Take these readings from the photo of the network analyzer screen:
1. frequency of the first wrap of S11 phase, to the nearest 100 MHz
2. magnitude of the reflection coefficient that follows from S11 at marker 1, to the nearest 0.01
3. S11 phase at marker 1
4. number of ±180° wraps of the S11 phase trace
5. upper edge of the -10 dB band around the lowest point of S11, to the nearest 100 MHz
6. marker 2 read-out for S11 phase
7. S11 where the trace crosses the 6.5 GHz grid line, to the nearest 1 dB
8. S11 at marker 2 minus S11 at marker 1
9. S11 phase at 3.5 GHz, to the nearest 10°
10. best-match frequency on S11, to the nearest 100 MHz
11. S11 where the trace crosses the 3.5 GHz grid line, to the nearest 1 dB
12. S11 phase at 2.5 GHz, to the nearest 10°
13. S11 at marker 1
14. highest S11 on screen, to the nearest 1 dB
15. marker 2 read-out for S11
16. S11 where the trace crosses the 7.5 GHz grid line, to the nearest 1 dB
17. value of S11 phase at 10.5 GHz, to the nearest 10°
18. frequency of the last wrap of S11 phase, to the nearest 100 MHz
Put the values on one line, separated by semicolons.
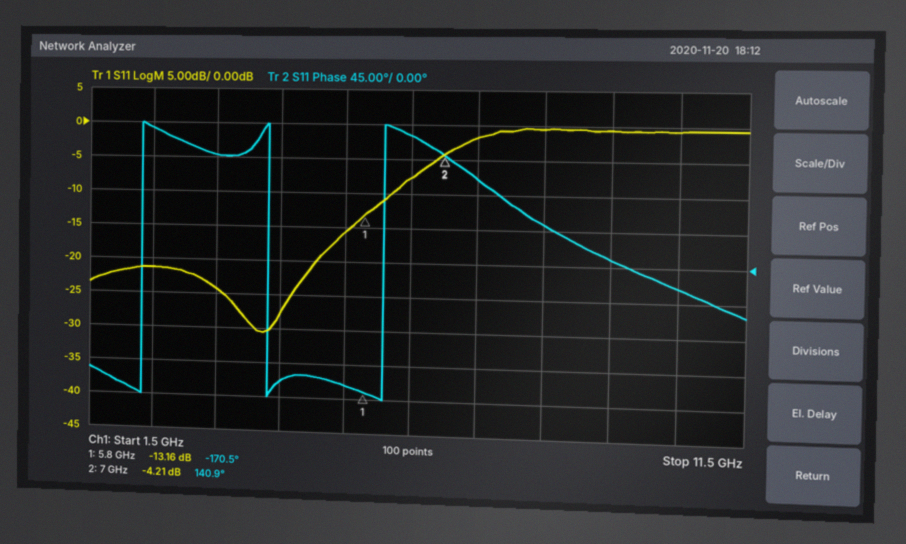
2.3 GHz; 0.22; -170.5°; 3; 6.2 GHz; 140.9°; -8 dB; 8.95 dB; 140°; 4.2 GHz; -24 dB; 170°; -13.16 dB; 0 dB; -4.21 dB; -2 dB; -30°; 6.1 GHz
